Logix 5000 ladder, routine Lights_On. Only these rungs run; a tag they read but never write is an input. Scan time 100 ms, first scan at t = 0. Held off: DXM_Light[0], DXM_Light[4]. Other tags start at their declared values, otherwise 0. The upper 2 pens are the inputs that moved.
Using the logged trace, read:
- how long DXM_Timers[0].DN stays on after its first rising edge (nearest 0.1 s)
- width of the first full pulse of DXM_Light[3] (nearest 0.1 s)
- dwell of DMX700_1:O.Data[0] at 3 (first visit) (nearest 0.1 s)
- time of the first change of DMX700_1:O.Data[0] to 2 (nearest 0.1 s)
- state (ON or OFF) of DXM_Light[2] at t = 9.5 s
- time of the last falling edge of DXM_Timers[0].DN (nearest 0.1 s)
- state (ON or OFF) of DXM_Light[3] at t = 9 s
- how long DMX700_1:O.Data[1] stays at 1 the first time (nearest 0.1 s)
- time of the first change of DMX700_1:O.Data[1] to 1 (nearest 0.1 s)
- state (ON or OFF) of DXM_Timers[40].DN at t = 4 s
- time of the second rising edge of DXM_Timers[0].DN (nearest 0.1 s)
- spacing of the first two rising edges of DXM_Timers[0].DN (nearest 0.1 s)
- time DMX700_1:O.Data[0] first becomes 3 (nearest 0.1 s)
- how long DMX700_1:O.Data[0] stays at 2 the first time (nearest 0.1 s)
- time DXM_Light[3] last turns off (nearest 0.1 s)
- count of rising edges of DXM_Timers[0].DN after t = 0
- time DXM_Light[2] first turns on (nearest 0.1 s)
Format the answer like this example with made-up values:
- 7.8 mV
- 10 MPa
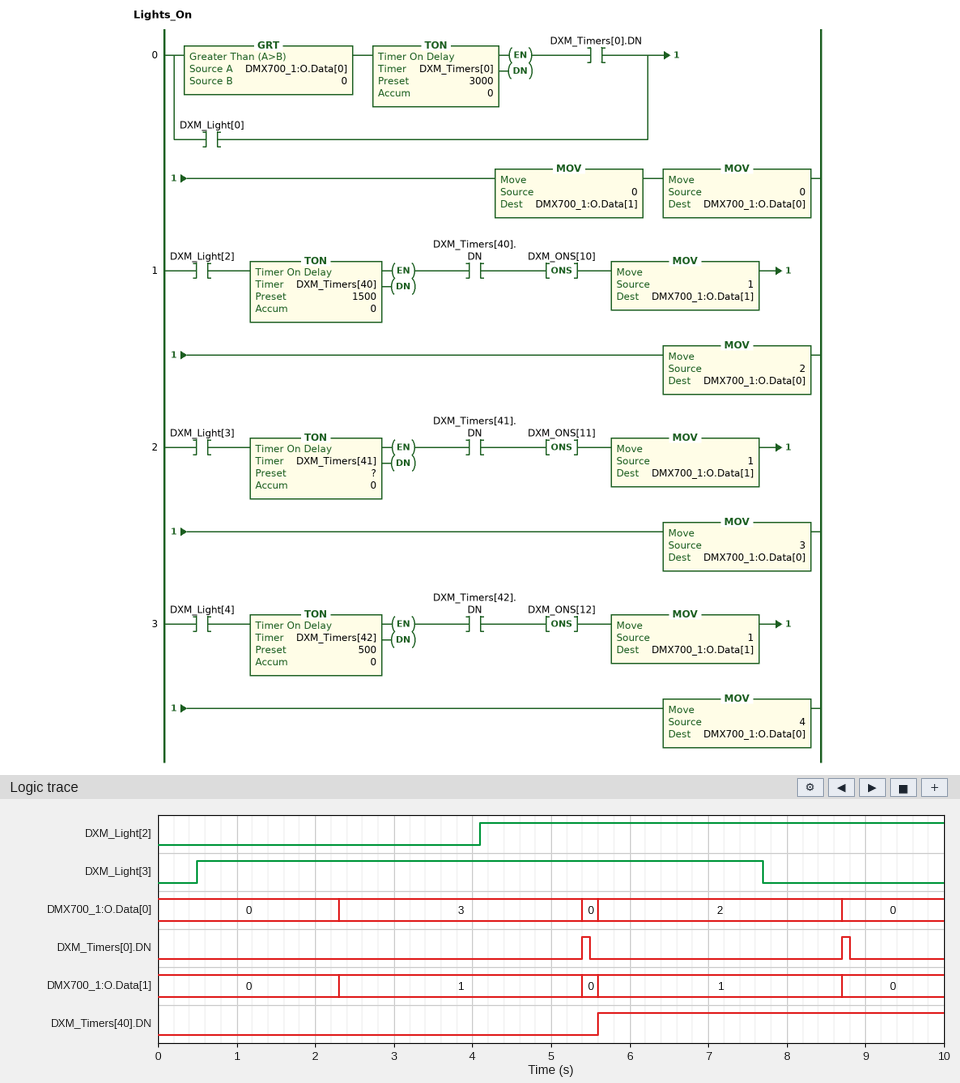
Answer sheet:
- 0.1 s
- 7.2 s
- 3.1 s
- 5.6 s
- ON
- 8.8 s
- OFF
- 3.1 s
- 2.3 s
- OFF
- 8.7 s
- 3.3 s
- 2.3 s
- 3.1 s
- 7.7 s
- 2
- 4.1 s
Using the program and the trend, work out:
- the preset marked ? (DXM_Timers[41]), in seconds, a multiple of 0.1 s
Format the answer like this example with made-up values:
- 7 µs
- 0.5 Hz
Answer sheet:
- 1.8 s
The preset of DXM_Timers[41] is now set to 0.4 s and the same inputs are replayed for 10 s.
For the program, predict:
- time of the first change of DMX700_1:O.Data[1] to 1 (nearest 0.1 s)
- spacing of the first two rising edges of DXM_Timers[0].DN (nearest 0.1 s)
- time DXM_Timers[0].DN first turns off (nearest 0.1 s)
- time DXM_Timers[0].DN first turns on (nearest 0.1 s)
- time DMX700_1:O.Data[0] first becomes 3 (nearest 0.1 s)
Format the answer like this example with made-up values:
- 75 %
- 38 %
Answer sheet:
- 0.9 s
- 4.7 s
- 4.1 s
- 4.0 s
- 0.9 s
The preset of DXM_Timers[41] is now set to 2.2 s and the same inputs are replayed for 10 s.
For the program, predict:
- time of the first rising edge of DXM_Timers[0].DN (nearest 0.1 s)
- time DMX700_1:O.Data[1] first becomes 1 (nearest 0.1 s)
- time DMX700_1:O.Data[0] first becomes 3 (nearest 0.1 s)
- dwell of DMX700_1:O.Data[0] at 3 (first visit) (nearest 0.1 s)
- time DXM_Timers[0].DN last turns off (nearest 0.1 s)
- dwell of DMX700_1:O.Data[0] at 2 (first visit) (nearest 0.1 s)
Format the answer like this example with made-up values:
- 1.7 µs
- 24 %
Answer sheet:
- 5.8 s
- 2.7 s
- 2.7 s
- 2.9 s
- 5.9 s
- 0.2 s
